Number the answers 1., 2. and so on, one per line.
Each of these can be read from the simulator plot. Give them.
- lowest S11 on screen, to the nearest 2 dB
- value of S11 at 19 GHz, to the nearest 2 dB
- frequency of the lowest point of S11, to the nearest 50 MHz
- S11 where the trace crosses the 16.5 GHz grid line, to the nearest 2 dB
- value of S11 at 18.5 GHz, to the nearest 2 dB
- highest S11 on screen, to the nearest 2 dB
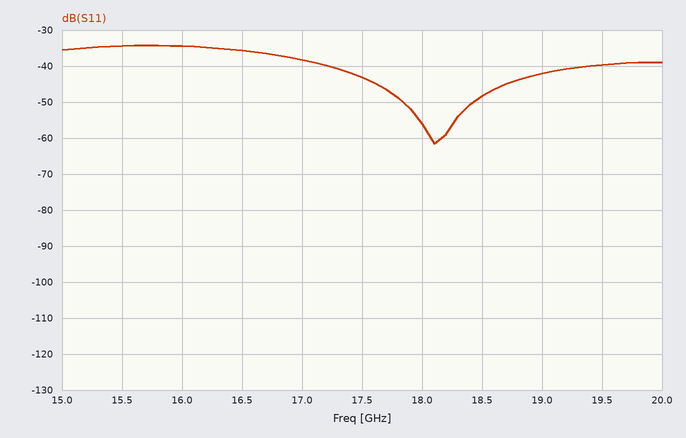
1. -62 dB
2. -42 dB
3. 18.10 GHz
4. -36 dB
5. -48 dB
6. -34 dB
